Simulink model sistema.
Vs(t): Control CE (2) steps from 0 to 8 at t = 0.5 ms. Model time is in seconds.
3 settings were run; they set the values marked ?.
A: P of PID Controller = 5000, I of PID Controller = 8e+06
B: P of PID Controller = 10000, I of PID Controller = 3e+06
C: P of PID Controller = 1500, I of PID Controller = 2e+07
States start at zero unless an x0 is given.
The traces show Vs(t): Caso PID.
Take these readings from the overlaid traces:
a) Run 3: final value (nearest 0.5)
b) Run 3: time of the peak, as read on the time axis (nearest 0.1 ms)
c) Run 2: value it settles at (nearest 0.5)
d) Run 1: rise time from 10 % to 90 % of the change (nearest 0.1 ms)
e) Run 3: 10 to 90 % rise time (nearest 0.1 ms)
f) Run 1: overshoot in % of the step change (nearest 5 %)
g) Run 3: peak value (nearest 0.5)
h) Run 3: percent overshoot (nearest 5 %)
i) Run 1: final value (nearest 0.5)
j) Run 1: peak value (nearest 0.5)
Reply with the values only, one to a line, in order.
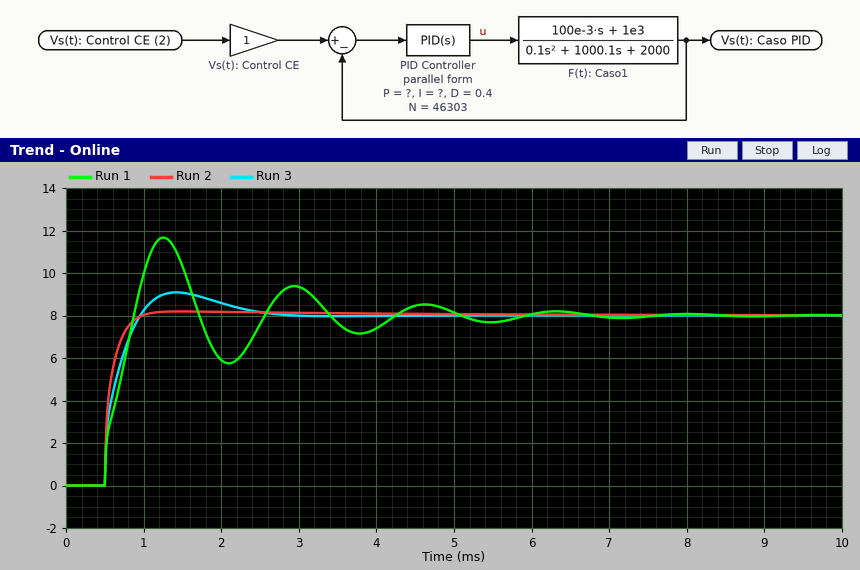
8.0
1.4 ms
8.0
0.3 ms
0.3 ms
45 %
9.0
15 %
8.0
11.5
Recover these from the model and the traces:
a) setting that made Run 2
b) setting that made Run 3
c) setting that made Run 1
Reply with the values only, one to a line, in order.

B
A
C
